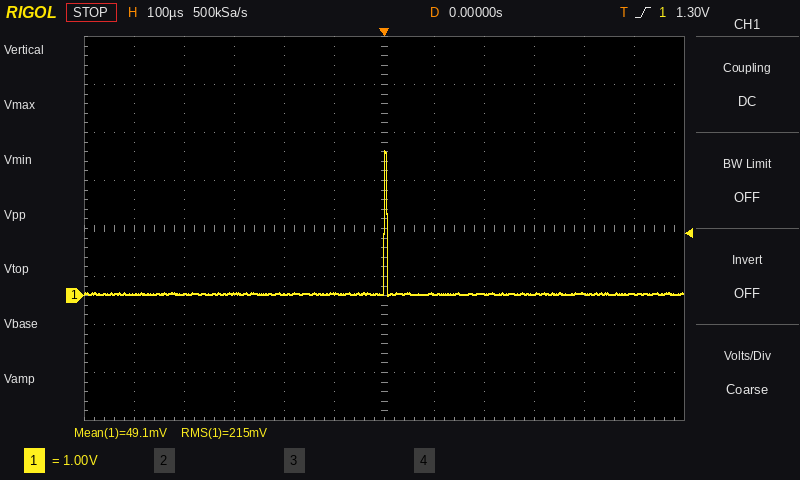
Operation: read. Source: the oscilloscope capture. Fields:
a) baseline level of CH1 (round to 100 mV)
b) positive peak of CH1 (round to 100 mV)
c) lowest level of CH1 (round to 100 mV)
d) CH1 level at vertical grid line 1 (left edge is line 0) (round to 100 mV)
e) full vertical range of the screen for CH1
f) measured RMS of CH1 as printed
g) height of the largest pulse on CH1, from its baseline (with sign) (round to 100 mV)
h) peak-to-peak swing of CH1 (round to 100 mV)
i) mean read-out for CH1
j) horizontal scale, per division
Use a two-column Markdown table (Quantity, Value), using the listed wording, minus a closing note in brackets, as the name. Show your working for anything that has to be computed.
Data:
| Quantity | Value |
|---|---|
| baseline level of CH1 | 0.0 V |
| positive peak of CH1 | 3.0 V |
| lowest level of CH1 | 0.0 V |
| CH1 level at vertical grid line 1 (left edge is line 0) | 0.0 V |
| full vertical range of the screen for CH1 | 8 V |
| measured RMS of CH1 as printed | 215 mV |
| height of the largest pulse on CH1, from its baseline (with sign) | 3.0 V − (0.0 V) = +3.0 V |
| peak-to-peak swing of CH1 | 3.0 V − (0.0 V) = 3.0 V |
| mean read-out for CH1 | 49.1 mV |
| horizontal scale, per division | 100 µs |
